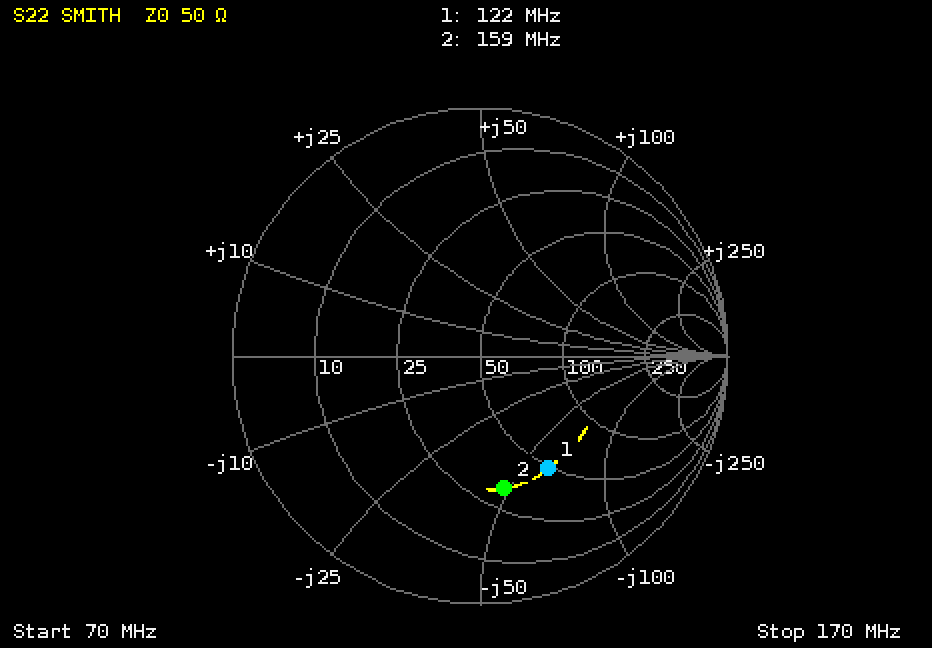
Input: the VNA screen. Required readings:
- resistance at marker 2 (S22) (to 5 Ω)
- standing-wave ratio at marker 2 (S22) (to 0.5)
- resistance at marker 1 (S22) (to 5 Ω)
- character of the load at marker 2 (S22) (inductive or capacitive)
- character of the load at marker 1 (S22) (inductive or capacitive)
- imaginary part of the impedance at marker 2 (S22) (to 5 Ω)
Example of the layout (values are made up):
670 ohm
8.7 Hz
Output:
30 Ω
3.5
50 Ω
capacitive
capacitive
-50 Ω
